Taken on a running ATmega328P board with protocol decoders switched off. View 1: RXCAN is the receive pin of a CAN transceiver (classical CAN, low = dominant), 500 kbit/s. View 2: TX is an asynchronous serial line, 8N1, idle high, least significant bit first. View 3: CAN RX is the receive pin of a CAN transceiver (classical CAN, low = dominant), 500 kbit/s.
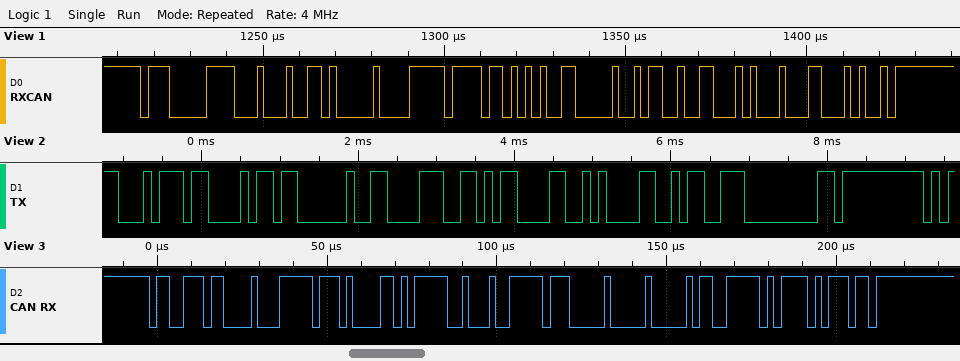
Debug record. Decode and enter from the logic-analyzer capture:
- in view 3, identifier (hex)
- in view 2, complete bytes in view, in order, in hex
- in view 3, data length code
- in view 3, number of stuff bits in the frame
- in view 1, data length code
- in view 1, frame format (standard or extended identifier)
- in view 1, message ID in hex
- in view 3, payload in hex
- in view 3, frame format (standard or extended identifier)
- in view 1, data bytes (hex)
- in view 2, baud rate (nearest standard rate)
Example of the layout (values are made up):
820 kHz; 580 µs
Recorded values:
0x676; 0x74 0x68 0x20 0x38 0x0D 0x0A 0x9A 0x00 0xFF; 8; 7; 8; standard; 0x707; FF 43 5F 44 FF 00 00 CF; standard; 9A 00 FF B5 4C 05 93 14; 9600 baud
